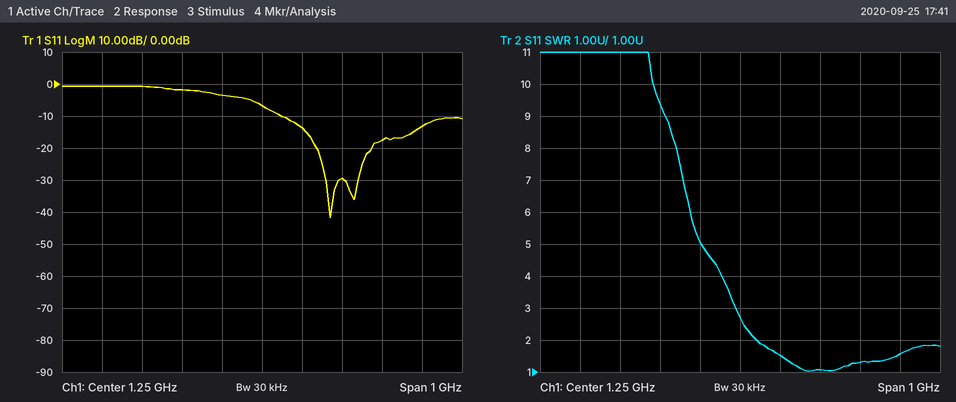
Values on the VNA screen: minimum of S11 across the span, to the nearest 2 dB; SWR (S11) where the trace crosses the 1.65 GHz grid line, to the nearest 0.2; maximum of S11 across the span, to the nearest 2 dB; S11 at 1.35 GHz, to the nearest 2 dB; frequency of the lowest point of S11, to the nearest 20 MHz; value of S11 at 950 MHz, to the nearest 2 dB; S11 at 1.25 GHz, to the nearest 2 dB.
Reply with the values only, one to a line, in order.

-42 dB
1.6
0 dB
-14 dB
1.42 GHz
0 dB
-6 dB
